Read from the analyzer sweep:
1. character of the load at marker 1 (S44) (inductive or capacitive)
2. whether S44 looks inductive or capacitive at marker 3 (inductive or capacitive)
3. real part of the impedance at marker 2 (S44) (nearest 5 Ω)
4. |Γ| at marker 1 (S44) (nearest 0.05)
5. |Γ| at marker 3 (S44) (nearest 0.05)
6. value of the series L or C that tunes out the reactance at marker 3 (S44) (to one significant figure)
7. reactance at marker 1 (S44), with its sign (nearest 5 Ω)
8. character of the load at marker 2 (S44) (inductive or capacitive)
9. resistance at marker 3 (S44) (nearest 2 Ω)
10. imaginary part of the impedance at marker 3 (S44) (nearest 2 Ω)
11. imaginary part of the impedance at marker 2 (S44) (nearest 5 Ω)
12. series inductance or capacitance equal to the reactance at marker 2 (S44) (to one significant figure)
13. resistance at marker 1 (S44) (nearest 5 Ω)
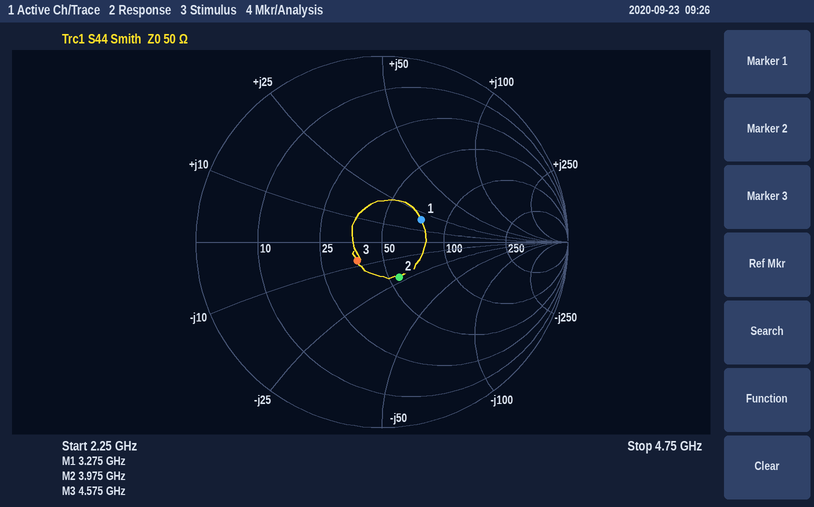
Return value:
inductive
capacitive
55 Ω
0.25
0.15
300 pH
+20 Ω
capacitive
38 Ω
-8 Ω
-20 Ω
2 pF
75 Ω
